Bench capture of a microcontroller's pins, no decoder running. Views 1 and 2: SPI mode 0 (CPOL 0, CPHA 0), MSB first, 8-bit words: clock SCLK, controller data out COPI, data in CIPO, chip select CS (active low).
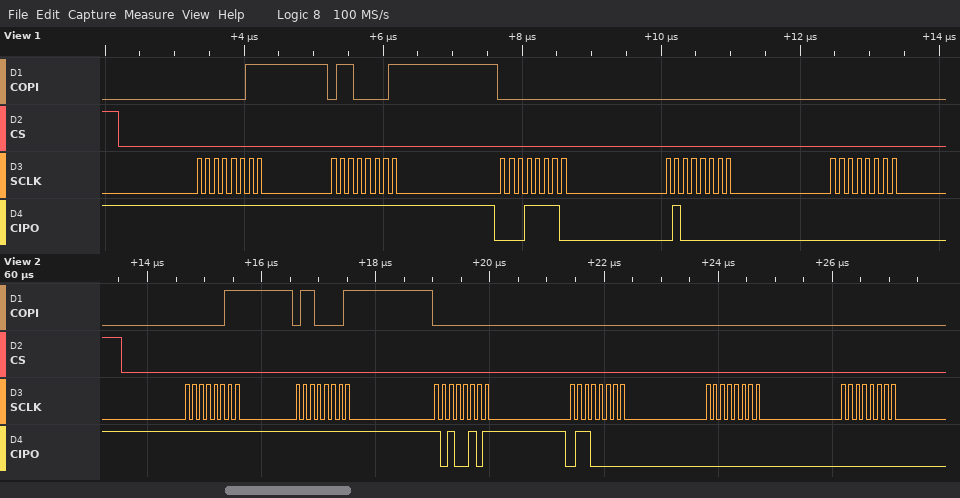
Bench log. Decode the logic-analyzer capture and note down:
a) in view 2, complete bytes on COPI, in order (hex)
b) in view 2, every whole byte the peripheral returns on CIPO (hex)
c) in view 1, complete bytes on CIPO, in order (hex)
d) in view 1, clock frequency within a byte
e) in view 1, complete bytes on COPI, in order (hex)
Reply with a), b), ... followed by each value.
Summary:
a) 03 61 00 00 00 00
b) FF FF A5 60 00 00
c) FF FF 1E 40 00
d) 8 MHz
e) 03 61 00 00 00
